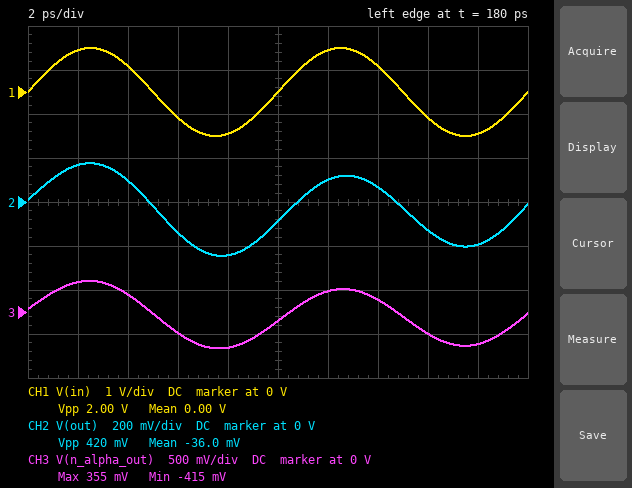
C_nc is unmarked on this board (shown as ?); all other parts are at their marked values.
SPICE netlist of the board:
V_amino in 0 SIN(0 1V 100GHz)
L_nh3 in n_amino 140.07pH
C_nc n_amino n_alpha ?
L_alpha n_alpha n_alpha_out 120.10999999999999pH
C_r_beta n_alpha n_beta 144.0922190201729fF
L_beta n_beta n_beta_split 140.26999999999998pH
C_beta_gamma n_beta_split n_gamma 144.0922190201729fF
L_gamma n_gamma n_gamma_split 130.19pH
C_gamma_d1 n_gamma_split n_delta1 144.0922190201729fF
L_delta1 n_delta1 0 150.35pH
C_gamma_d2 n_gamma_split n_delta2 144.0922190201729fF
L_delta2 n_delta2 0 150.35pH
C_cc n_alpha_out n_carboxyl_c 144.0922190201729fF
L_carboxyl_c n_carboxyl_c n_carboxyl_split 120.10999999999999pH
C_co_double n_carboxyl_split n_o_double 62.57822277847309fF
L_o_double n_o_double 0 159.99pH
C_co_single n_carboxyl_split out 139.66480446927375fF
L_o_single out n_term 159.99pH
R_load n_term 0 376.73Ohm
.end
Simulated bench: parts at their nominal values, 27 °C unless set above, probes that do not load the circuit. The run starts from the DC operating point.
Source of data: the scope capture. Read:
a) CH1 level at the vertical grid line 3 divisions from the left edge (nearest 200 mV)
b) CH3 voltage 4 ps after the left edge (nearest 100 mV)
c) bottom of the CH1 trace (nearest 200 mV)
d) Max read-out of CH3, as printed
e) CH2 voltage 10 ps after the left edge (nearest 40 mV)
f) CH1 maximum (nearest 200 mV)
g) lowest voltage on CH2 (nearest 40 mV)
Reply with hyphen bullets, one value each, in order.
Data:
- -600 mV
- 200 mV
- -1.0 V
- 355 mV
- -80 mV
- 1.0 V
- -240 mV
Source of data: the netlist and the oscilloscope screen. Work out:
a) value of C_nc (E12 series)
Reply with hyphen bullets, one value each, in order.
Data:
- 560 fF
